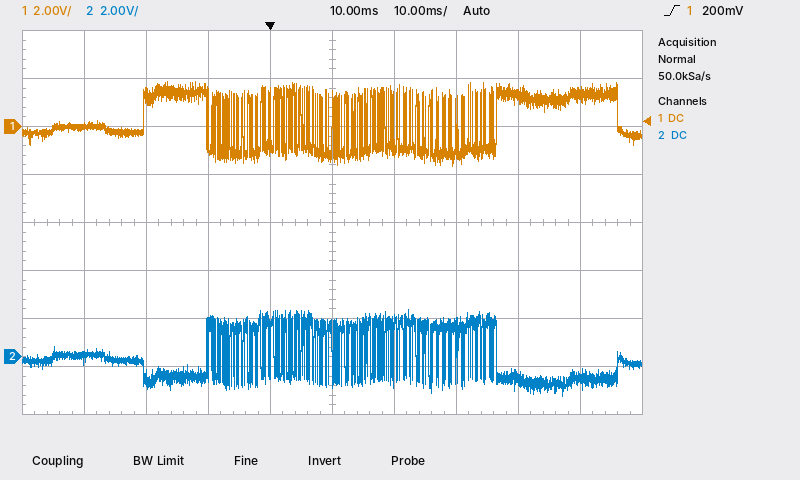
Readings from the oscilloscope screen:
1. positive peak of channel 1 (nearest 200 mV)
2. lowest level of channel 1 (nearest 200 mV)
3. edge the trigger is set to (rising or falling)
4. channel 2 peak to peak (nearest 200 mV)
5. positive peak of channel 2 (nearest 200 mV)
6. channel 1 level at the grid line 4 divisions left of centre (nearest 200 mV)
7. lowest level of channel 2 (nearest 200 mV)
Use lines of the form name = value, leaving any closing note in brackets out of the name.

positive peak of channel 1 = 1.8 V
lowest level of channel 1 = -1.6 V
edge the trigger is set to = rising
channel 2 peak to peak = 3.6 V
positive peak of channel 2 = 2.0 V
channel 1 level at the grid line 4 divisions left of centre = 0.0 V
lowest level of channel 2 = -1.6 V
